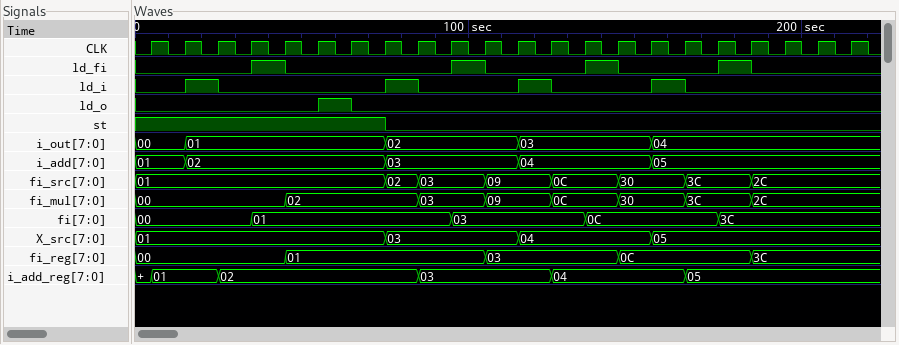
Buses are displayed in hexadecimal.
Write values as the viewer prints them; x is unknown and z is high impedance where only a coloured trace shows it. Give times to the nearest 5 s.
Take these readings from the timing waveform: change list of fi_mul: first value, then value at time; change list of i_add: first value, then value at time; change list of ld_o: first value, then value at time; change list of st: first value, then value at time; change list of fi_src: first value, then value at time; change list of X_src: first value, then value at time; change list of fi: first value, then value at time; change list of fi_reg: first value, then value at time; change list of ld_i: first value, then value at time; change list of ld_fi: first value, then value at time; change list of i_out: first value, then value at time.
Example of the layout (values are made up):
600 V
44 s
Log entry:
00, 02 at 45 s, 03 at 85 s, 09 at 105 s, 0C at 125 s, 30 at 145 s, 3C at 165 s, 2C at 185 s
01, 02 at 15 s, 03 at 75 s, 04 at 115 s, 05 at 155 s
0, 1 at 55 s, 0 at 65 s
1, 0 at 75 s
01, 02 at 75 s, 03 at 85 s, 09 at 105 s, 0C at 125 s, 30 at 145 s, 3C at 165 s, 2C at 185 s
01, 03 at 75 s, 04 at 115 s, 05 at 155 s
00, 01 at 35 s, 03 at 95 s, 0C at 135 s, 3C at 175 s
00, 01 at 45 s, 03 at 105 s, 0C at 145 s, 3C at 185 s
0, 1 at 15 s, 0 at 25 s, 1 at 75 s, 0 at 85 s, 1 at 115 s, 0 at 125 s, 1 at 155 s, 0 at 165 s
0, 1 at 35 s, 0 at 45 s, 1 at 95 s, 0 at 105 s, 1 at 135 s, 0 at 145 s, 1 at 175 s, 0 at 185 s
00, 01 at 15 s, 02 at 75 s, 03 at 115 s, 04 at 155 s
